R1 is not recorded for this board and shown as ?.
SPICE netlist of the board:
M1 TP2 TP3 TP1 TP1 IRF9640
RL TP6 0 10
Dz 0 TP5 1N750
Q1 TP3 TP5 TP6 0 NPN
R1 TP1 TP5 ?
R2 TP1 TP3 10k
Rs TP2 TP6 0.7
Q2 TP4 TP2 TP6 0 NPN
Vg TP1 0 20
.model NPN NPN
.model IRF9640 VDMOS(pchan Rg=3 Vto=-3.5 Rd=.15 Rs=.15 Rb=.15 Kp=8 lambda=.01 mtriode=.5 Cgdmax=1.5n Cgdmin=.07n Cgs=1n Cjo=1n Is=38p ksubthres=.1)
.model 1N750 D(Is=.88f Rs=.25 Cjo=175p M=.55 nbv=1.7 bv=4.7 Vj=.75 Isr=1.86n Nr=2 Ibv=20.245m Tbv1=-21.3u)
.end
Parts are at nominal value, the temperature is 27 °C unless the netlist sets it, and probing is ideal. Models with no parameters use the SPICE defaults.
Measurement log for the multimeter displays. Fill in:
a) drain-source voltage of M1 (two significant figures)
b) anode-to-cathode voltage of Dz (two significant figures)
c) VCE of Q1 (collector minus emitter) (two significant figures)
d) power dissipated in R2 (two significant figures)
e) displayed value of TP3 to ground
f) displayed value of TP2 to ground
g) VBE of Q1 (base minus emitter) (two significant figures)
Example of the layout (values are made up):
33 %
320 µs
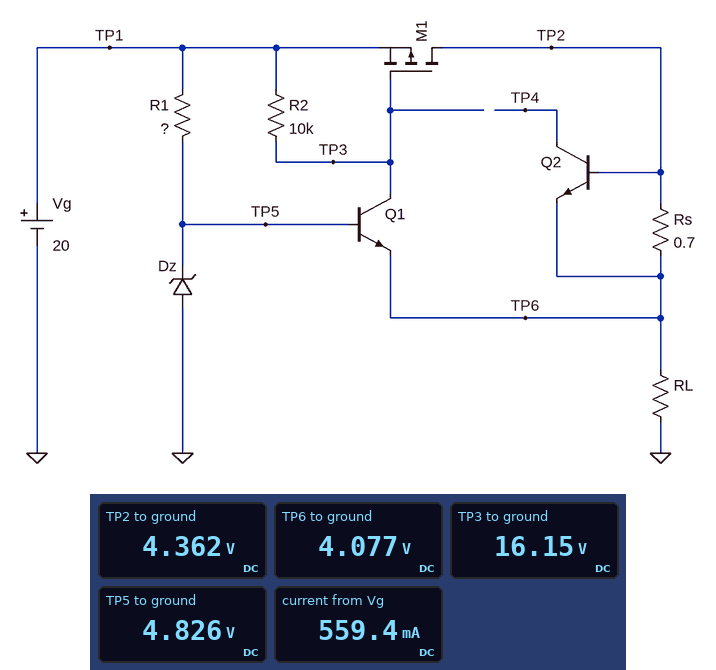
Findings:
-16 V
-4.8 V
12 V
1.5 mW
16.15 V
4.362 V
750 mV
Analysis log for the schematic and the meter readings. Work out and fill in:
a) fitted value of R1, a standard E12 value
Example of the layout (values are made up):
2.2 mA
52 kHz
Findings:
100 Ω
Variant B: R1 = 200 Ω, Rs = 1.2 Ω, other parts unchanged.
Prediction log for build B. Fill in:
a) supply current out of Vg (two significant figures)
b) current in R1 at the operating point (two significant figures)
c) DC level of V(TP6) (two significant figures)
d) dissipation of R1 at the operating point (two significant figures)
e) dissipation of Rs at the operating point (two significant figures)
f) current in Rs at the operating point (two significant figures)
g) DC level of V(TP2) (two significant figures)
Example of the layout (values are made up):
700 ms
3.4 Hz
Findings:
480 mA
76 mA
4.0 V
1.2 W
190 mW
400 mA
4.5 V
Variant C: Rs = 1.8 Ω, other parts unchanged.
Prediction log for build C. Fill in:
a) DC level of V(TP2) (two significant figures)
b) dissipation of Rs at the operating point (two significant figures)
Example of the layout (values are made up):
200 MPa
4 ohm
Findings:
4.8 V
300 mW
